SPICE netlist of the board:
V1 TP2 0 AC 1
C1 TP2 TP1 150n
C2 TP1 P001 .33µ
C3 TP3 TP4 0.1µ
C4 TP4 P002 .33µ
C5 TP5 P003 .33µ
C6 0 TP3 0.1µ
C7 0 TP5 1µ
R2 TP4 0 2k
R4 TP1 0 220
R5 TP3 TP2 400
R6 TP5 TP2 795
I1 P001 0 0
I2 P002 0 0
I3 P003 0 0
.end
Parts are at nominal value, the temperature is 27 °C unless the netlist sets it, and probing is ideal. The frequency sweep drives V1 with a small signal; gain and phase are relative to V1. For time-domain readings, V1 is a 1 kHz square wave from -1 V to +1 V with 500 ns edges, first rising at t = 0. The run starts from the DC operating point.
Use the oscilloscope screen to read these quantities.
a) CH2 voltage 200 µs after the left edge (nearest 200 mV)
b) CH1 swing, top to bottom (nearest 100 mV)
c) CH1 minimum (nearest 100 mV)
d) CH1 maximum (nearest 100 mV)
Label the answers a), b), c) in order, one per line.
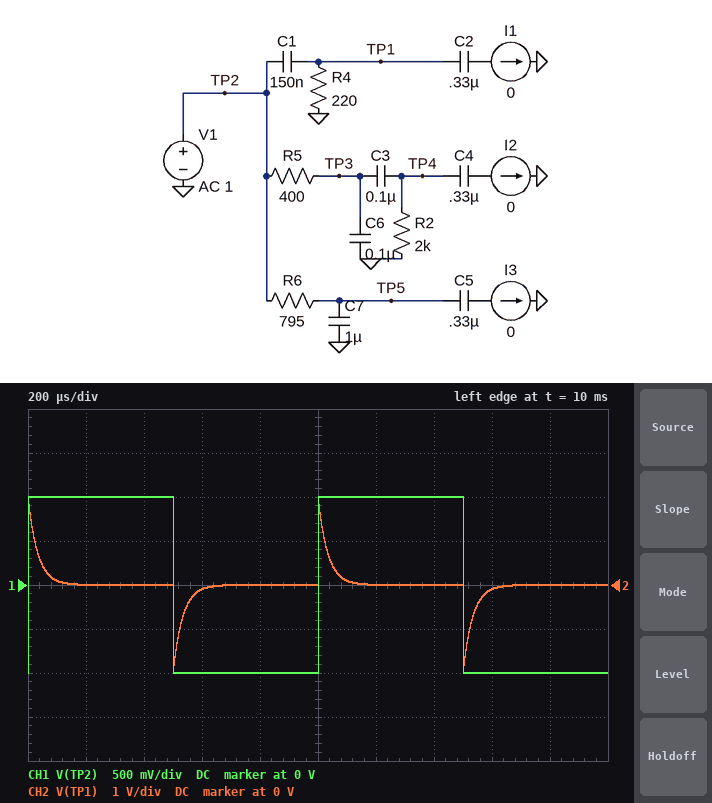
a) 0 V
b) 2.0 V
c) -1.0 V
d) 1.0 V
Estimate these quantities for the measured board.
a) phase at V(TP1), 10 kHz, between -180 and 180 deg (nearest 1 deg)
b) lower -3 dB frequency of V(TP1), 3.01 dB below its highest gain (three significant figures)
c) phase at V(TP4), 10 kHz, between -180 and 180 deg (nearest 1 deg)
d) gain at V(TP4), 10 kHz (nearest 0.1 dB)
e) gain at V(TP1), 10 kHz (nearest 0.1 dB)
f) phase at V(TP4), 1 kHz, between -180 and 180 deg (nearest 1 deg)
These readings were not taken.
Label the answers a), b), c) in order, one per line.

a) 26 deg
b) 4.82 kHz
c) -60 deg
d) -9.0 dB
e) -0.9 dB
f) 21 deg
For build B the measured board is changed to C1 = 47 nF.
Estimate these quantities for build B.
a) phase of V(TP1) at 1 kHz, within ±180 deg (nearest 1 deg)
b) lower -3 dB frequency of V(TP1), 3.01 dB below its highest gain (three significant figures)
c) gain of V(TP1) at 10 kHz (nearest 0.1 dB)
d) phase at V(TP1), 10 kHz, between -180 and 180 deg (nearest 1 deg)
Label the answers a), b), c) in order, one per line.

a) 86 deg
b) 15.4 kHz
c) -5.3 dB
d) 57 deg
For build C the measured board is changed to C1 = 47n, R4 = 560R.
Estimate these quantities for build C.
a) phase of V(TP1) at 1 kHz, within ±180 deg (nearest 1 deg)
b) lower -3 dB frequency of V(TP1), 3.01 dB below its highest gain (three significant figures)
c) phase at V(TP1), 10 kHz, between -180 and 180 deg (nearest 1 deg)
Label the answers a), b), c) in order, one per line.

a) 81 deg
b) 6.05 kHz
c) 31 deg
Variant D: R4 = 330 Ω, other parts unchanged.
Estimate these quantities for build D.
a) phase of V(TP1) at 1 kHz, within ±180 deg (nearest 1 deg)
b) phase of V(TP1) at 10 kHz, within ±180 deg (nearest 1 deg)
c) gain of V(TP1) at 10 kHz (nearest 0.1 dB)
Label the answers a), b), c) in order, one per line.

a) 73 deg
b) 18 deg
c) -0.4 dB
